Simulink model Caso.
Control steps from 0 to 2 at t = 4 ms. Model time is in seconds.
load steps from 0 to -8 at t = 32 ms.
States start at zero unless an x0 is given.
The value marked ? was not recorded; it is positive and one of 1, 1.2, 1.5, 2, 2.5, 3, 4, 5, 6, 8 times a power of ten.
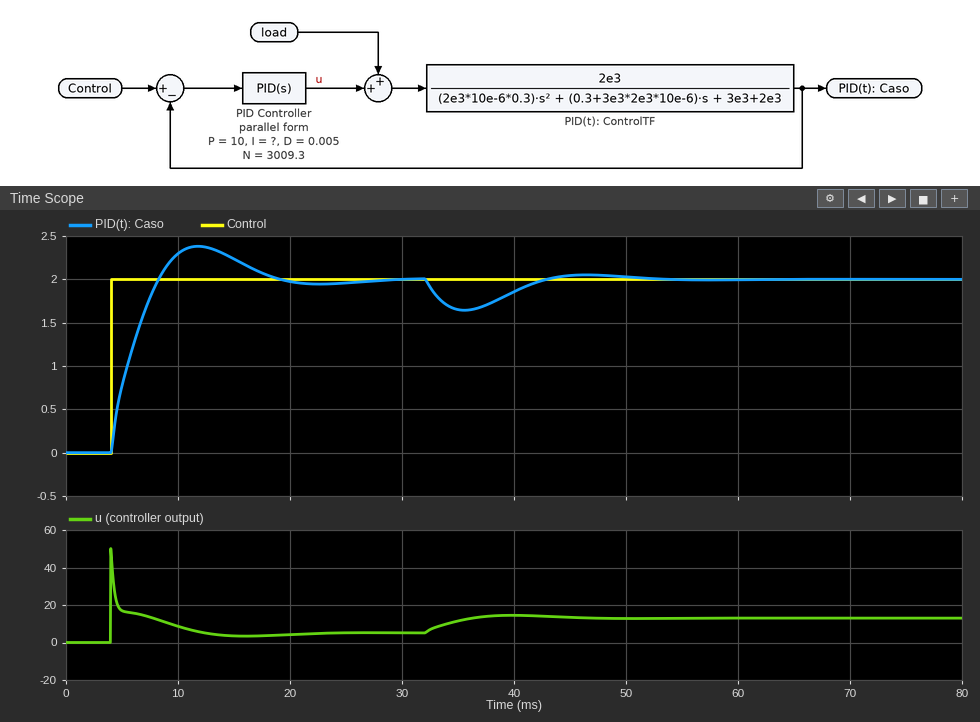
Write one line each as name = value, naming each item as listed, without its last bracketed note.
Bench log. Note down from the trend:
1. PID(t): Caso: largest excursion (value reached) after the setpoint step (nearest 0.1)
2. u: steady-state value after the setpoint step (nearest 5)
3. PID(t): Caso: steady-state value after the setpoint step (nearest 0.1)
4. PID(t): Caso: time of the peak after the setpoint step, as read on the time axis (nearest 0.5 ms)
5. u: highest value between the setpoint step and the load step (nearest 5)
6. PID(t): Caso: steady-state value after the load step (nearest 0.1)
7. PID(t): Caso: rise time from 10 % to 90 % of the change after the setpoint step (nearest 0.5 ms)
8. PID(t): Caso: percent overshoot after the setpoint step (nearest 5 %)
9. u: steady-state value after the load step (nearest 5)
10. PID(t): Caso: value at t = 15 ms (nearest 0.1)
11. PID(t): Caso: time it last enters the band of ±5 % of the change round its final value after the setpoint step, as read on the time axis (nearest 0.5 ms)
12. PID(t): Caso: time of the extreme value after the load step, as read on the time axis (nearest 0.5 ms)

PID(t): Caso: largest excursion (value reached) after the setpoint step = 2.4
u: steady-state value after the setpoint step = 5
PID(t): Caso: steady-state value after the setpoint step = 2.0
PID(t): Caso: time of the peak after the setpoint step, as read on the time axis = 12.0 ms
u: highest value between the setpoint step and the load step = 50
PID(t): Caso: steady-state value after the load step = 2.0
PID(t): Caso: rise time from 10 % to 90 % of the change after the setpoint step = 3.5 ms
PID(t): Caso: percent overshoot after the setpoint step = 20 %
u: steady-state value after the load step = 15
PID(t): Caso: value at t = 15 ms = 2.2
PID(t): Caso: time it last enters the band of ±5 % of the change round its final value after the setpoint step, as read on the time axis = 17.0 ms
PID(t): Caso: time of the extreme value after the load step, as read on the time axis = 35.5 ms
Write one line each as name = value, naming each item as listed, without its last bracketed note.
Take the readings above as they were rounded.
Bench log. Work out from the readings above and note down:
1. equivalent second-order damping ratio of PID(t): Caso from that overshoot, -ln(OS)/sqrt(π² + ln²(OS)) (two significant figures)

equivalent second-order damping ratio of PID(t): Caso from that overshoot, -ln(OS)/sqrt(π² + ln²(OS)) = 0.46
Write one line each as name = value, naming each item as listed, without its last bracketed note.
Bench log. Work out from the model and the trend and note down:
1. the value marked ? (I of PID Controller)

the value marked ? = 4000
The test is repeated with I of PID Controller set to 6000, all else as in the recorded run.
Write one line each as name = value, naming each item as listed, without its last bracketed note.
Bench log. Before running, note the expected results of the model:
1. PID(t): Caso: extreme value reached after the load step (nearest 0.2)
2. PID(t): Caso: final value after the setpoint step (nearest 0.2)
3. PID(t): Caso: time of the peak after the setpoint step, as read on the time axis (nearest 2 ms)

PID(t): Caso: extreme value reached after the load step = 1.6
PID(t): Caso: final value after the setpoint step = 2.0
PID(t): Caso: time of the peak after the setpoint step, as read on the time axis = 10 ms
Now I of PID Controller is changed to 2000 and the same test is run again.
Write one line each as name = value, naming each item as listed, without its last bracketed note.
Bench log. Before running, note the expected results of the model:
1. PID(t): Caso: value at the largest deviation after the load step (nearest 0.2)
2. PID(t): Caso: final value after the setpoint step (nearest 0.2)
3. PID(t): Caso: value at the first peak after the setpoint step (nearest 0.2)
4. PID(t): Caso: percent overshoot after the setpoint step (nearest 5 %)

PID(t): Caso: value at the largest deviation after the load step = 1.6
PID(t): Caso: final value after the setpoint step = 2.0
PID(t): Caso: value at the first peak after the setpoint step = 2.2
PID(t): Caso: percent overshoot after the setpoint step = 10 %
